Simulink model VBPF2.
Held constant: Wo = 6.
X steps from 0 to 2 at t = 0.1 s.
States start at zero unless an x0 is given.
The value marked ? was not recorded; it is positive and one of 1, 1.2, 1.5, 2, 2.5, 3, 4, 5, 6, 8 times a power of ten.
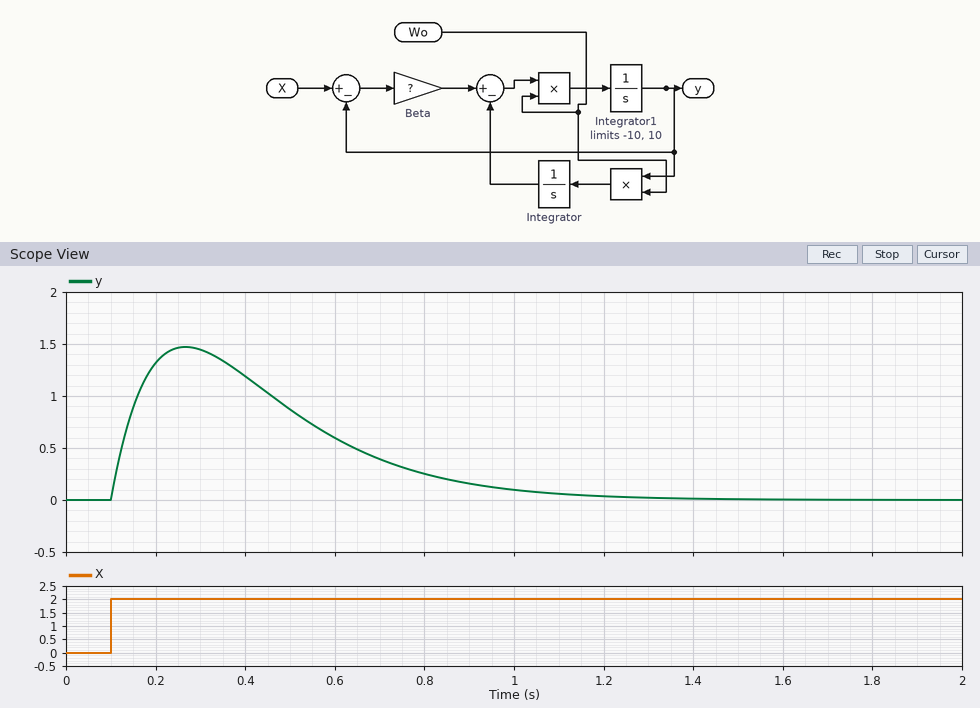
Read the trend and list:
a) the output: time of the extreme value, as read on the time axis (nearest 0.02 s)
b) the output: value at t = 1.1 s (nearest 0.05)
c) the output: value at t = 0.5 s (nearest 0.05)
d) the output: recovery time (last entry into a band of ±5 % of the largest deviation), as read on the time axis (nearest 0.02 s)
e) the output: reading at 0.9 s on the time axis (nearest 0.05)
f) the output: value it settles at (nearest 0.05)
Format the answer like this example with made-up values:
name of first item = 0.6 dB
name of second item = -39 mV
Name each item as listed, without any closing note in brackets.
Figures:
the output: time of the extreme value, as read on the time axis = 0.26 s
the output: value at t = 1.1 s = 0.05
the output: value at t = 0.5 s = 0.85
the output: recovery time (last entry into a band of ±5 % of the largest deviation), as read on the time axis = 1.06 s
the output: reading at 0.9 s on the time axis = 0.15
the output: value it settles at = 0.00
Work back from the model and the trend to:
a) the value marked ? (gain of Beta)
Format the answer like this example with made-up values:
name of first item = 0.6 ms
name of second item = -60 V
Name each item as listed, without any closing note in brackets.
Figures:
the value marked ? = 2
